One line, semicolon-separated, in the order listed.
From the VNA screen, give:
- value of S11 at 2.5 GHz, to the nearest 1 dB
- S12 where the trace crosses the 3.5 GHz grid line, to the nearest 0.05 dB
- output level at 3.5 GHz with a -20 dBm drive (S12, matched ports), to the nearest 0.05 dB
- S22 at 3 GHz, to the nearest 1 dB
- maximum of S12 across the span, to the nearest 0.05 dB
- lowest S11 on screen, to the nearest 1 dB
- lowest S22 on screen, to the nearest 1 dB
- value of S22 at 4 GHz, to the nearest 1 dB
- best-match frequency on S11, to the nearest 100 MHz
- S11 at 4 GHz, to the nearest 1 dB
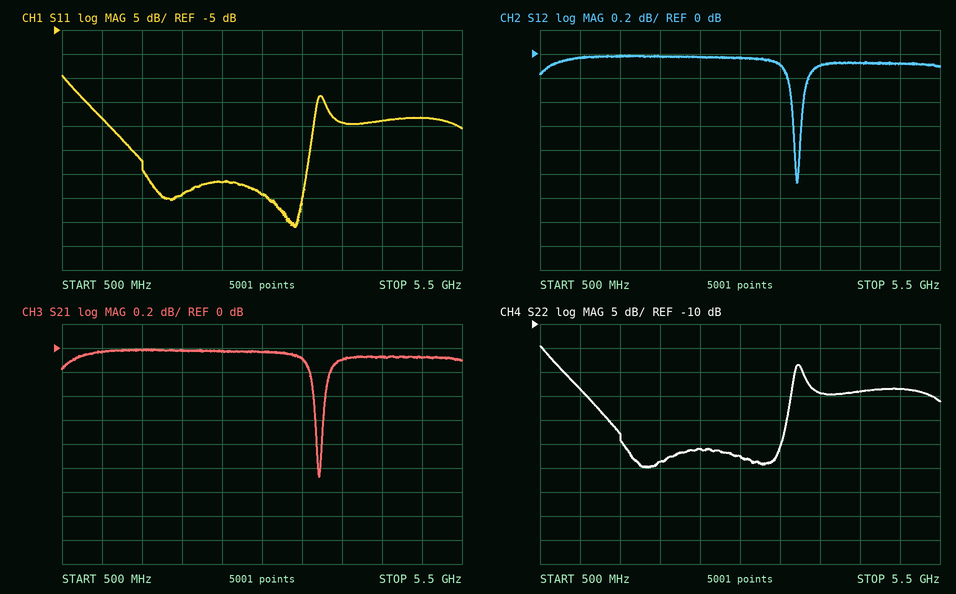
-37 dB; -0.10 dB; -20.10 dBm; -38 dB; 0.00 dB; -46 dB; -40 dB; -24 dB; 3.4 GHz; -24 dB
